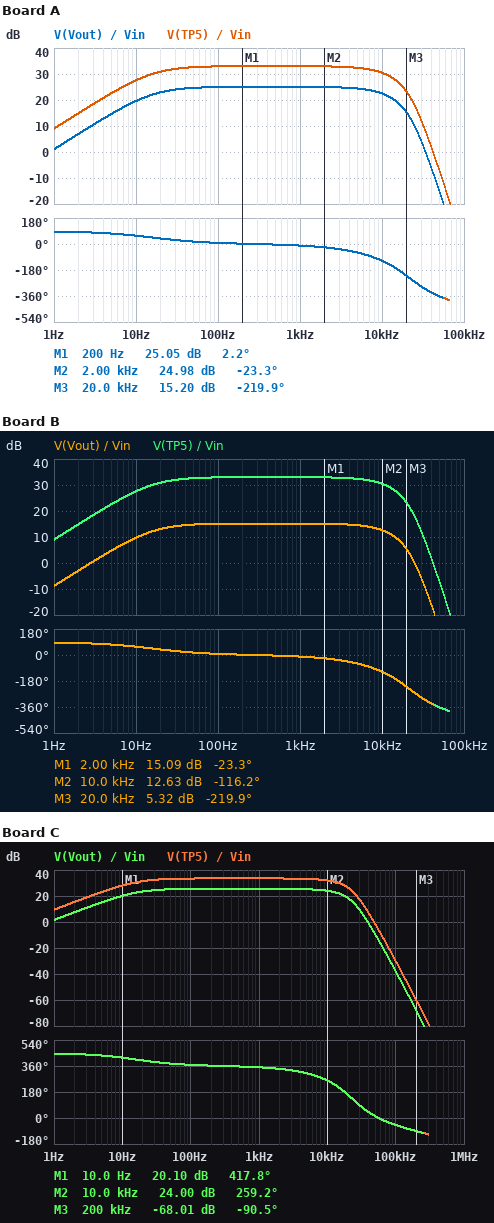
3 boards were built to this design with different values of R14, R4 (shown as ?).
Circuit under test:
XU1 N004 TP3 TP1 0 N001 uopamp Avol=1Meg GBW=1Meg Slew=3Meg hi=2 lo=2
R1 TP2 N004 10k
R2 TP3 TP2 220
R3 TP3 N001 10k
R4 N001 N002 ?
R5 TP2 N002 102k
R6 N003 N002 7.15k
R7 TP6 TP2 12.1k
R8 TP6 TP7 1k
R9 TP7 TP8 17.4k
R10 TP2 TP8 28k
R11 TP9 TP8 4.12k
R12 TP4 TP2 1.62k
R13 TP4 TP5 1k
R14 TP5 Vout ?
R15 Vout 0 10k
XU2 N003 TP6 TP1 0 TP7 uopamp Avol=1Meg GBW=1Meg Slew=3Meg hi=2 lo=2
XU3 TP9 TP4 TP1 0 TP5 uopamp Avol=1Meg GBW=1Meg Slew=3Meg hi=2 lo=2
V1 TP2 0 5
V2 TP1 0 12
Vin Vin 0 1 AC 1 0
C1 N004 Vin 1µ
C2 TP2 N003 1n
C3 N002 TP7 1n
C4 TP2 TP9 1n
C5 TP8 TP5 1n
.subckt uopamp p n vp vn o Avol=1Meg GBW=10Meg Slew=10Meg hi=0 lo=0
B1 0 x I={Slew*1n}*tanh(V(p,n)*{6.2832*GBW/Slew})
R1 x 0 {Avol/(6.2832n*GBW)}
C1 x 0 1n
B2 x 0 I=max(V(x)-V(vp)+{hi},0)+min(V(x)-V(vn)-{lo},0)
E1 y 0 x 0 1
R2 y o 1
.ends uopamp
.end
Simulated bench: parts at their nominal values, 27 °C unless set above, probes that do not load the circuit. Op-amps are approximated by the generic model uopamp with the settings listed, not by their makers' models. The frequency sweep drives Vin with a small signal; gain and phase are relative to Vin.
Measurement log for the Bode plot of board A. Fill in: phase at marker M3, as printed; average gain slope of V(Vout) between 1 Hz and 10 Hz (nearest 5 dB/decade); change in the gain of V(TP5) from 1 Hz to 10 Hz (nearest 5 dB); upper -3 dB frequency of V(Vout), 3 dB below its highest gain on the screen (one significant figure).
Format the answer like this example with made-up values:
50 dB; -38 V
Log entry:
-219.9 deg; 20 dB/decade; 20 dB; 10 kHz
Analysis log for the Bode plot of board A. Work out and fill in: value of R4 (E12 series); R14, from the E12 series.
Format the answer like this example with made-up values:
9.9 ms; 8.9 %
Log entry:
12 kΩ; 15 kΩ
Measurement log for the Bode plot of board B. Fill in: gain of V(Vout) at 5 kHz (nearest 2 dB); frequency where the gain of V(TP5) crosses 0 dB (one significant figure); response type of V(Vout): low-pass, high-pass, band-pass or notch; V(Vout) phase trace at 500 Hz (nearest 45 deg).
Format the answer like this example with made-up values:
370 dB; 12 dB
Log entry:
14 dB; 40 kHz; band-pass; 0 deg
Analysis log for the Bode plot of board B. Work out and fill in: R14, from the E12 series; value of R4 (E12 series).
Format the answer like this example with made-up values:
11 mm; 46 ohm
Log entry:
68 kΩ; 12 kΩ
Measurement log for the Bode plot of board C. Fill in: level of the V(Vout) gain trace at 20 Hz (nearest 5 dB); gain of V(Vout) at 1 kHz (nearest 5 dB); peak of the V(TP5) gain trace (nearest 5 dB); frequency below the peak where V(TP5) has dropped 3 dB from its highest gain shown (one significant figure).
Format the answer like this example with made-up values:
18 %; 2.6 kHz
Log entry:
25 dB; 25 dB; 35 dB; 20 Hz
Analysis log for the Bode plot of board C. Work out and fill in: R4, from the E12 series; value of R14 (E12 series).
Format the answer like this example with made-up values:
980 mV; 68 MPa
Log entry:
5.6 kΩ; 15 kΩ
